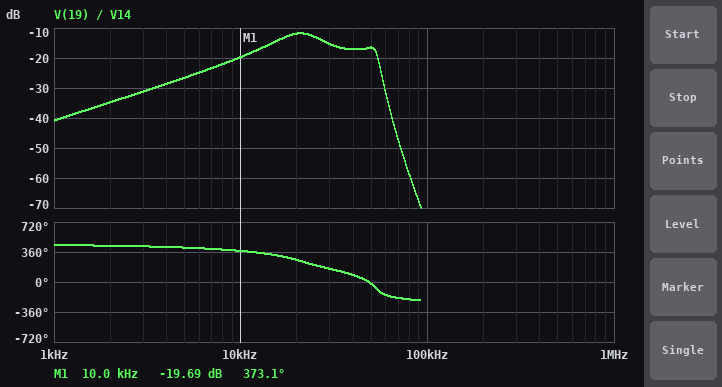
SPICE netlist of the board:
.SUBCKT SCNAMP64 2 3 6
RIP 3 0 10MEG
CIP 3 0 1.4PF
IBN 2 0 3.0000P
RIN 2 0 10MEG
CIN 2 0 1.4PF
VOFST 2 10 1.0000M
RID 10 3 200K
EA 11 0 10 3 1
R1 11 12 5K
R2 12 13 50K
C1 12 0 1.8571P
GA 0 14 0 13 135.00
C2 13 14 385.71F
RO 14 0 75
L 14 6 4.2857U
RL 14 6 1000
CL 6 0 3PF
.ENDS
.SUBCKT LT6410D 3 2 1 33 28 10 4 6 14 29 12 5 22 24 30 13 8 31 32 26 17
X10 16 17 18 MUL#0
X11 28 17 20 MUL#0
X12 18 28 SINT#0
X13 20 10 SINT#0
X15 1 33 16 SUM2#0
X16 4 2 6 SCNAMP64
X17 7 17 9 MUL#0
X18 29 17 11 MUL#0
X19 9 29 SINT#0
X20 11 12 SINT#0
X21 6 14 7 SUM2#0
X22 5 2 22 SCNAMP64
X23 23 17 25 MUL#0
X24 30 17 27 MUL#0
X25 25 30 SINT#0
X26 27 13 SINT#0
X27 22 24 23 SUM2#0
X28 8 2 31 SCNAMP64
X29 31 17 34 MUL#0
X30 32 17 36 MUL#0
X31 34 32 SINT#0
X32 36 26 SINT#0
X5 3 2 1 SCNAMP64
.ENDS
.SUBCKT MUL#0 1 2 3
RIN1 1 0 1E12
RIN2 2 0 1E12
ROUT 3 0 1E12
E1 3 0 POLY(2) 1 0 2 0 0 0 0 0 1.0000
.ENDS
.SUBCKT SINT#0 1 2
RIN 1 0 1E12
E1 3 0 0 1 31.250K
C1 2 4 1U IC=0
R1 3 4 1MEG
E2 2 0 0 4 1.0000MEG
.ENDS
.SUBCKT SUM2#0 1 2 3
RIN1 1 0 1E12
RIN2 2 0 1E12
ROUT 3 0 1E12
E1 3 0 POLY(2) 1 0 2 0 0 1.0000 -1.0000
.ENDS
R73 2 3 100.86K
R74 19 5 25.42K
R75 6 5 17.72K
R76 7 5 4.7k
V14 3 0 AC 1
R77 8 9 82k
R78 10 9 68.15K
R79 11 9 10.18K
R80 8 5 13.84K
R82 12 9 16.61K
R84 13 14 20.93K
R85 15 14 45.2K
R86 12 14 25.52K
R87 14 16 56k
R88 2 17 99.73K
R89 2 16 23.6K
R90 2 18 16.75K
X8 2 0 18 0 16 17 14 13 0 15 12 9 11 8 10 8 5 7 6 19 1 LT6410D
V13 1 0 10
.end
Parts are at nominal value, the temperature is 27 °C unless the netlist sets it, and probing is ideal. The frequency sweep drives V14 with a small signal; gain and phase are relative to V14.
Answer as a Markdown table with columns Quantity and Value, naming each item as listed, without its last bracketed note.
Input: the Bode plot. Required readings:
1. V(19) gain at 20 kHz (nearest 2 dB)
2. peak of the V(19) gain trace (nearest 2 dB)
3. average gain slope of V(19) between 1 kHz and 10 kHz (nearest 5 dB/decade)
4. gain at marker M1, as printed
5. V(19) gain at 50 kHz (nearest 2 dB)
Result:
| Quantity | Value |
|---|---|
| V(19) gain at 20 kHz | -12 dB |
| peak of the V(19) gain trace | -12 dB |
| average gain slope of V(19) between 1 kHz and 10 kHz | 20 dB/decade |
| gain at marker M1, as printed | -19.69 dB |
| V(19) gain at 50 kHz | -16 dB |
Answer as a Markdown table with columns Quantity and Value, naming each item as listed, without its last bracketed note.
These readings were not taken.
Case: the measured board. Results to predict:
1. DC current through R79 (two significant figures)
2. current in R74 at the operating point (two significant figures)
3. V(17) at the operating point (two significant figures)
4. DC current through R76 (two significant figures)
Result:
| Quantity | Value |
|---|---|
| DC current through R79 | 110 nA |
| current in R74 at the operating point | 350 nA |
| V(17) at the operating point | 12 mV |
| DC current through R76 | 210 nA |
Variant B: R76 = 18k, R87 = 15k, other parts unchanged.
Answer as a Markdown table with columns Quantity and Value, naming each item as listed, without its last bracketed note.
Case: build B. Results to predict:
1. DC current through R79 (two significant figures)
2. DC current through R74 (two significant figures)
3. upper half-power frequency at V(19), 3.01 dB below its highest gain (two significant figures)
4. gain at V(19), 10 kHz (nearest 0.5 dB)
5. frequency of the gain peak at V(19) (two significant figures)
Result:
| Quantity | Value |
|---|---|
| DC current through R79 | 170 nA |
| DC current through R74 | 240 nA |
| upper half-power frequency at V(19), 3.01 dB below its highest gain | 54 kHz |
| gain at V(19), 10 kHz | -9.5 dB |
| frequency of the gain peak at V(19) | 51 kHz |
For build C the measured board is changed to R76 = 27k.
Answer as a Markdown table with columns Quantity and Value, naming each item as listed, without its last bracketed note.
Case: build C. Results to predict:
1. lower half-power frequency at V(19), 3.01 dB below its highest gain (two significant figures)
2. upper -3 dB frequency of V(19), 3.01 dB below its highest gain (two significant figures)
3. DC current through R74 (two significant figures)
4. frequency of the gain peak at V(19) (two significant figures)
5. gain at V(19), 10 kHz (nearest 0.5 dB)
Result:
| Quantity | Value |
|---|---|
| lower half-power frequency at V(19), 3.01 dB below its highest gain | 43 kHz |
| upper -3 dB frequency of V(19), 3.01 dB below its highest gain | 54 kHz |
| DC current through R74 | 170 nA |
| frequency of the gain peak at V(19) | 51 kHz |
| gain at V(19), 10 kHz | -21.5 dB |
